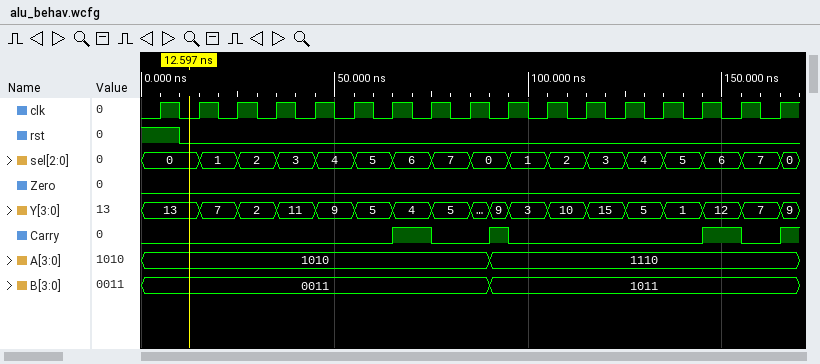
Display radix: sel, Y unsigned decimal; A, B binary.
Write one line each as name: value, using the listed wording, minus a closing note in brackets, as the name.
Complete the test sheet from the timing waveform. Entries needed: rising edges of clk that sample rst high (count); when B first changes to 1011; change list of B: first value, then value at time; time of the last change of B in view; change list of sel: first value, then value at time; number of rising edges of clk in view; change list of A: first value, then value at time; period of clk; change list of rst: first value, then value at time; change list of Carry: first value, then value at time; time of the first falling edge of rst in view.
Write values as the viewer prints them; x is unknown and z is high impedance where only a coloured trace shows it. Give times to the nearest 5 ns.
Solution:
rising edges of clk that sample rst high: 1
when B first changes to 1011: 90 ns
change list of B: first value, then value at time: 0011, 1011 at 90 ns
time of the last change of B in view: 90 ns
change list of sel: first value, then value at time: 0, 1 at 15 ns, 2 at 25 ns, 3 at 35 ns, 4 at 45 ns, 5 at 55 ns, 6 at 65 ns, 7 at 75 ns, 0 at 85 ns, 1 at 95 ns, 2 at 105 ns, 3 at 115 ns, 4 at 125 ns, 5 at 135 ns, 6 at 145 ns, 7 at 155 ns, 0 at 165 ns
number of rising edges of clk in view: 17
change list of A: first value, then value at time: 1010, 1110 at 90 ns
period of clk: 10 ns
change list of rst: first value, then value at time: 1, 0 at 10 ns
change list of Carry: first value, then value at time: 0, 1 at 65 ns, 0 at 75 ns, 1 at 90 ns, 0 at 95 ns, 1 at 145 ns, 0 at 155 ns, 1 at 165 ns
time of the first falling edge of rst in view: 10 ns
